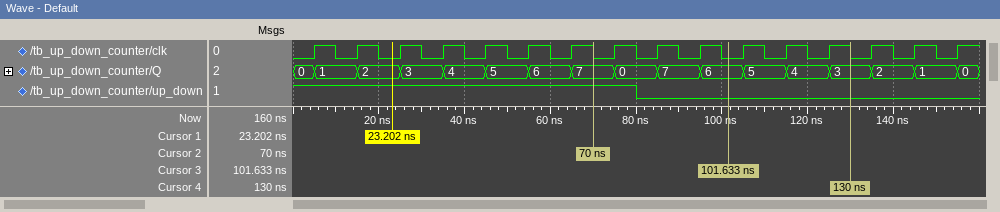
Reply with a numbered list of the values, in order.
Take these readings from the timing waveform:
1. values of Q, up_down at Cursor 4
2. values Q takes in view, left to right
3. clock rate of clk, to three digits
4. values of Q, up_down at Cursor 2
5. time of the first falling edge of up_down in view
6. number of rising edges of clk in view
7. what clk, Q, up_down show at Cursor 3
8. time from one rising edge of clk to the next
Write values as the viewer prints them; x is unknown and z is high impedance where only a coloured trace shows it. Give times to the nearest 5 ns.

1. Q=3, up_down=0
2. 0, 1, 2, 3, 4, 5, 6, 7, 0, 7, 6, 5, 4, 3, 2, 1, 0
3. 100 MHz
4. Q=7, up_down=1
5. 80 ns
6. 16
7. clk=0, Q=6, up_down=0
8. 10 ns
